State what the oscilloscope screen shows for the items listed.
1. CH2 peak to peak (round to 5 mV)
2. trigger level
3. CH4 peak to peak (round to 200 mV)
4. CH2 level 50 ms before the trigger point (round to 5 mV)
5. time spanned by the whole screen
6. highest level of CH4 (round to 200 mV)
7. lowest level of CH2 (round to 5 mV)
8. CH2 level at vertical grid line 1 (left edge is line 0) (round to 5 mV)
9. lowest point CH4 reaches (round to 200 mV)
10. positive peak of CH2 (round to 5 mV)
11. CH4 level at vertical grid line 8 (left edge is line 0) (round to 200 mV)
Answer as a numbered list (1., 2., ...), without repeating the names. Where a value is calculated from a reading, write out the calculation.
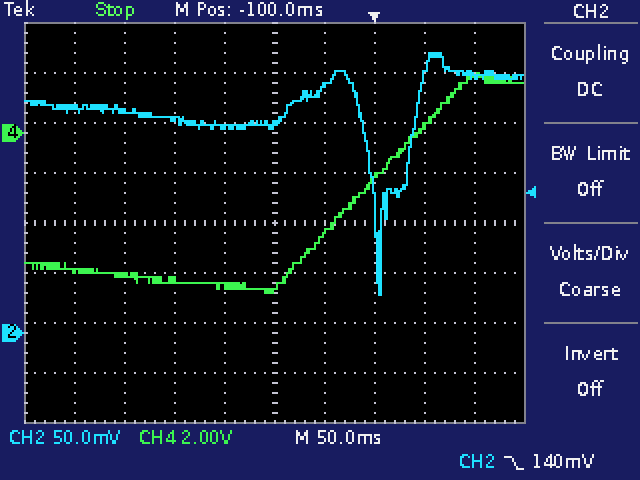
1. 280 mV − (40 mV) = 240 mV
2. 140 mV
3. 2.4 V − (-6.4 V) = 8.8 V
4. 245 mV
5. 500 ms
6. 2.4 V
7. 40 mV
8. 225 mV
9. -6.4 V
10. 280 mV
11. 200 mV
